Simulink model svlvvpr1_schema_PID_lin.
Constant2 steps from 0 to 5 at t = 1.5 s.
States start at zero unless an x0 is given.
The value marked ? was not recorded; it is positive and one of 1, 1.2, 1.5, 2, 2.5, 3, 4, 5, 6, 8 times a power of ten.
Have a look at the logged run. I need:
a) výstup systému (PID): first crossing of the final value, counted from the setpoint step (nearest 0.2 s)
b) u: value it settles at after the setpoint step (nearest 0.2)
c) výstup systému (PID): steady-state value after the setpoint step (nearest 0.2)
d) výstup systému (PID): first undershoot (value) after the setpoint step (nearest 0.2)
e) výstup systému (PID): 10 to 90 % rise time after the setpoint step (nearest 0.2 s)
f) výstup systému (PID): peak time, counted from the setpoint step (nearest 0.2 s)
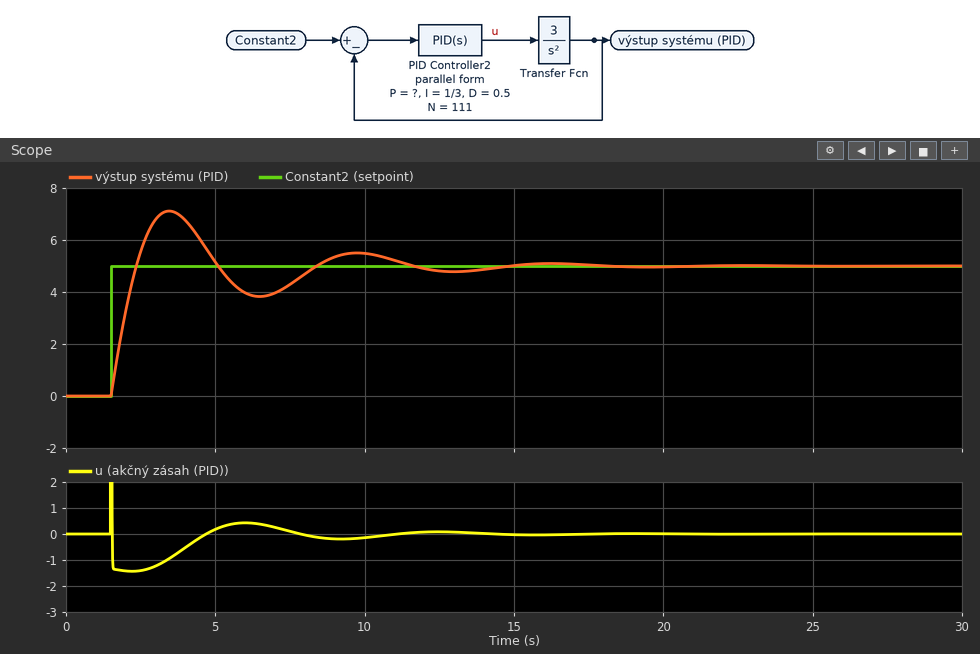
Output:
0.8 s
0.0
5.0
3.8
0.6 s
2.0 s
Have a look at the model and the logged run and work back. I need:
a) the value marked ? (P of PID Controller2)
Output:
0.5
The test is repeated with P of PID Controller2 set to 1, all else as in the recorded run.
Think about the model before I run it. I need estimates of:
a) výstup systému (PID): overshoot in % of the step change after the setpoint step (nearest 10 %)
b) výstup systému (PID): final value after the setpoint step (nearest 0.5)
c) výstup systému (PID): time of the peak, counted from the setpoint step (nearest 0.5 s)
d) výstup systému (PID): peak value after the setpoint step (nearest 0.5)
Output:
40 %
5.0
1.5 s
7.0
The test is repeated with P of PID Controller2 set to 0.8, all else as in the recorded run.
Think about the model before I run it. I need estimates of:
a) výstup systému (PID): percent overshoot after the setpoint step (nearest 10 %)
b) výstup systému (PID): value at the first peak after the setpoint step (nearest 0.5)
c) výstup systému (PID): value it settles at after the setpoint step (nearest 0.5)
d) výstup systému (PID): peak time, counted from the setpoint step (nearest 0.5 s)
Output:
40 %
7.0
5.0
1.5 s
